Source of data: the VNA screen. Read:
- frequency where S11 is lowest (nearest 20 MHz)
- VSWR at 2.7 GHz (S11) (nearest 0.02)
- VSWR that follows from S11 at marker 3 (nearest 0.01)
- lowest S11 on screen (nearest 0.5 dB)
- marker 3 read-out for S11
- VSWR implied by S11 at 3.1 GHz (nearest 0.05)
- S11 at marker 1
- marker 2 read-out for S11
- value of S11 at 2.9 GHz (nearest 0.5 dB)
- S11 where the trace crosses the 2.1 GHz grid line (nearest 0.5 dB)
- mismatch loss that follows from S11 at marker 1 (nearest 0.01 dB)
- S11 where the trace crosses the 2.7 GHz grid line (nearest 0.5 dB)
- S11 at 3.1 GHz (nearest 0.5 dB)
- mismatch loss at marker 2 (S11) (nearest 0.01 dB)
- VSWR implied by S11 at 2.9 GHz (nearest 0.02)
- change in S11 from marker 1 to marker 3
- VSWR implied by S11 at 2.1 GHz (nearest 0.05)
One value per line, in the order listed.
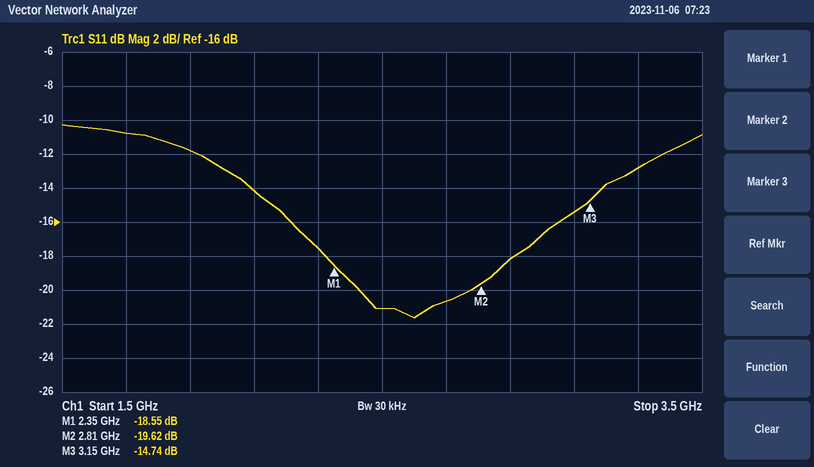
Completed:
2.60 GHz
1.20
1.45
-21.5 dB
-14.74 dB
1.40
-18.55 dB
-19.62 dB
-18.0 dB
-14.0 dB
0.06 dB
-20.5 dB
-15.5 dB
0.05 dB
1.28
3.81 dB
1.50
